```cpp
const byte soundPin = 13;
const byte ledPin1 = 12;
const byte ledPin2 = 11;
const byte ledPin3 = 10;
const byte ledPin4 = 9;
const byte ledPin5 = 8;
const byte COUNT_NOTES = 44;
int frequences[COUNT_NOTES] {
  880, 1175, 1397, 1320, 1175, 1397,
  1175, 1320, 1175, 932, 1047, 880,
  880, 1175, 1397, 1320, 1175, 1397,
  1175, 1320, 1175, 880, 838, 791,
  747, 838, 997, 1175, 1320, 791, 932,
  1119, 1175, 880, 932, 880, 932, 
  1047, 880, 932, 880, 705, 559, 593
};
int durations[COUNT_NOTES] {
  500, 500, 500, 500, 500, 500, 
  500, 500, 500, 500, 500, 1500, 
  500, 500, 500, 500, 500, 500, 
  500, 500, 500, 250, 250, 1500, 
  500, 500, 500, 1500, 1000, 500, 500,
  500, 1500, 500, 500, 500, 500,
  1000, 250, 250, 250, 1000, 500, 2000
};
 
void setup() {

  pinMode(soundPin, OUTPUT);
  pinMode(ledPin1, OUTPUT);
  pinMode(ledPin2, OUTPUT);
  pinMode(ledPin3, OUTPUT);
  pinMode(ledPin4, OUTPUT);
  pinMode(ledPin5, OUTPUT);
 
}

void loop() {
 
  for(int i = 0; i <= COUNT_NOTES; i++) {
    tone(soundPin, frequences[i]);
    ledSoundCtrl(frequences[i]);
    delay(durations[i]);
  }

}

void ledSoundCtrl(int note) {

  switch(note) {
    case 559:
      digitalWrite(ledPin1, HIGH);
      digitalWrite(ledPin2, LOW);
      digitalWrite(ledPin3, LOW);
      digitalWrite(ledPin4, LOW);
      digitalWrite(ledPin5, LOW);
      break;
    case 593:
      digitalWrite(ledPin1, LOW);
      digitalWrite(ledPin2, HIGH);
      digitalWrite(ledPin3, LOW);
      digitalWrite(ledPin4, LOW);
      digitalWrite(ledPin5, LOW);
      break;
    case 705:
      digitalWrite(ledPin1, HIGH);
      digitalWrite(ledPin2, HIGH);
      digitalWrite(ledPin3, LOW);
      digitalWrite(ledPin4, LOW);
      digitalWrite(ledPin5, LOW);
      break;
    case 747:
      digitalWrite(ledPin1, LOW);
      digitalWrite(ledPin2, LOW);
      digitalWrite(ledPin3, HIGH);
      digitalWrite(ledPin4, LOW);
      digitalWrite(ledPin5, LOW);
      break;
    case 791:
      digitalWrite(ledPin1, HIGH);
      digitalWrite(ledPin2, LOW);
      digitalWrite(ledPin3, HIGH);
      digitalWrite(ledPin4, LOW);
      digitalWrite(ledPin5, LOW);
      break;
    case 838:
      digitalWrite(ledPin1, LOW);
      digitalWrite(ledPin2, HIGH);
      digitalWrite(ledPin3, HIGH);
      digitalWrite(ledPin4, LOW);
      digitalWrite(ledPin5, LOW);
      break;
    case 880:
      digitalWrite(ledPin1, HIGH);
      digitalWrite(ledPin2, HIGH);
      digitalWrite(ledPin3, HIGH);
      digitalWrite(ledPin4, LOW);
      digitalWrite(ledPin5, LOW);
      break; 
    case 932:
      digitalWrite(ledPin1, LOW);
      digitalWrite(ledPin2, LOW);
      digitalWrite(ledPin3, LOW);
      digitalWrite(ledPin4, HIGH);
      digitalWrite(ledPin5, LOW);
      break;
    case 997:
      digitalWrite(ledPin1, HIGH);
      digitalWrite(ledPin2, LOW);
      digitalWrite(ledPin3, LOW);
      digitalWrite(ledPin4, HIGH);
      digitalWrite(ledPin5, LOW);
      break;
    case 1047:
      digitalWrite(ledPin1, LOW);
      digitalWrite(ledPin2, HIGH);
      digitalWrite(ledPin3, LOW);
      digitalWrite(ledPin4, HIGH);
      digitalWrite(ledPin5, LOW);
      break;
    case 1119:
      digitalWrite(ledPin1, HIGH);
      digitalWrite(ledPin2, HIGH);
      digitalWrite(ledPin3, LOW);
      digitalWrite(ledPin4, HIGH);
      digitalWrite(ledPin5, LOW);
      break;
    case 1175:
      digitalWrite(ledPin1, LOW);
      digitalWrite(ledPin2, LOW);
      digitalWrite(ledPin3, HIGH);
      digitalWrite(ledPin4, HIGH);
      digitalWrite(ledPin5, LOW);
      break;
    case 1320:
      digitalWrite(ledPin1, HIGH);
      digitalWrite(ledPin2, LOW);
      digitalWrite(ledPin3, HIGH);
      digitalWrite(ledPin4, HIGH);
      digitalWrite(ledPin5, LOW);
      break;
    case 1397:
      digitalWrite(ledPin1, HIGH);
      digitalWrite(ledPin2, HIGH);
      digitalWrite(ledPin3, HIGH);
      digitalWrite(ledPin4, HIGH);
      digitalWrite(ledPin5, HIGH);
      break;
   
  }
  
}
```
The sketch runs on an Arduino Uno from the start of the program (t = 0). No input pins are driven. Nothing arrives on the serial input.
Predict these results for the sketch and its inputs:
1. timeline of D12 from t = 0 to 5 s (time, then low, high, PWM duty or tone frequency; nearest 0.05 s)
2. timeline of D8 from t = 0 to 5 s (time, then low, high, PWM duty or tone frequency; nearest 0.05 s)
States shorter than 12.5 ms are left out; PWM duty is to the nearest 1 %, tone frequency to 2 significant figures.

0 s high; 0.5 s low; 1 s high; 2 s low; 2.5 s high; 3 s low; 3.5 s high; 4 s low
0 s low; 1 s high; 1.5 s low; 2.5 s high; 3 s low
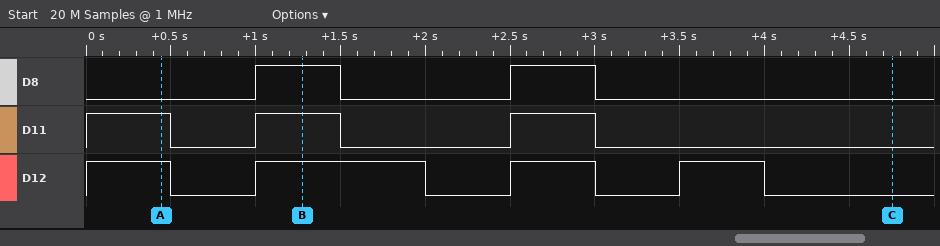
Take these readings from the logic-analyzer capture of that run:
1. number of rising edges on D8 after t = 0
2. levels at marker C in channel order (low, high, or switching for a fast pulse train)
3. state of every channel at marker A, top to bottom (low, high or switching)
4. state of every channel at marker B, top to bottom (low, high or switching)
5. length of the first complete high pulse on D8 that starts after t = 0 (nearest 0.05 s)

2
D8 low, D11 low, D12 low
D8 low, D11 high, D12 high
D8 high, D11 high, D12 high
0.50 s
